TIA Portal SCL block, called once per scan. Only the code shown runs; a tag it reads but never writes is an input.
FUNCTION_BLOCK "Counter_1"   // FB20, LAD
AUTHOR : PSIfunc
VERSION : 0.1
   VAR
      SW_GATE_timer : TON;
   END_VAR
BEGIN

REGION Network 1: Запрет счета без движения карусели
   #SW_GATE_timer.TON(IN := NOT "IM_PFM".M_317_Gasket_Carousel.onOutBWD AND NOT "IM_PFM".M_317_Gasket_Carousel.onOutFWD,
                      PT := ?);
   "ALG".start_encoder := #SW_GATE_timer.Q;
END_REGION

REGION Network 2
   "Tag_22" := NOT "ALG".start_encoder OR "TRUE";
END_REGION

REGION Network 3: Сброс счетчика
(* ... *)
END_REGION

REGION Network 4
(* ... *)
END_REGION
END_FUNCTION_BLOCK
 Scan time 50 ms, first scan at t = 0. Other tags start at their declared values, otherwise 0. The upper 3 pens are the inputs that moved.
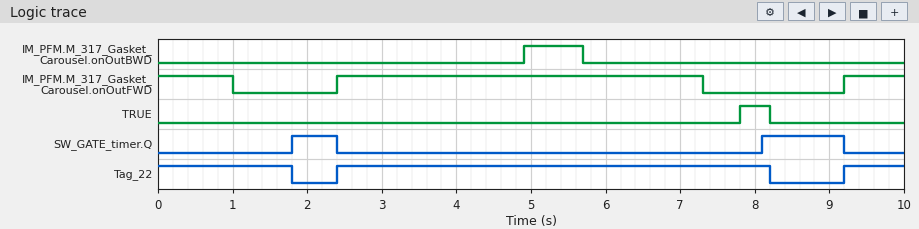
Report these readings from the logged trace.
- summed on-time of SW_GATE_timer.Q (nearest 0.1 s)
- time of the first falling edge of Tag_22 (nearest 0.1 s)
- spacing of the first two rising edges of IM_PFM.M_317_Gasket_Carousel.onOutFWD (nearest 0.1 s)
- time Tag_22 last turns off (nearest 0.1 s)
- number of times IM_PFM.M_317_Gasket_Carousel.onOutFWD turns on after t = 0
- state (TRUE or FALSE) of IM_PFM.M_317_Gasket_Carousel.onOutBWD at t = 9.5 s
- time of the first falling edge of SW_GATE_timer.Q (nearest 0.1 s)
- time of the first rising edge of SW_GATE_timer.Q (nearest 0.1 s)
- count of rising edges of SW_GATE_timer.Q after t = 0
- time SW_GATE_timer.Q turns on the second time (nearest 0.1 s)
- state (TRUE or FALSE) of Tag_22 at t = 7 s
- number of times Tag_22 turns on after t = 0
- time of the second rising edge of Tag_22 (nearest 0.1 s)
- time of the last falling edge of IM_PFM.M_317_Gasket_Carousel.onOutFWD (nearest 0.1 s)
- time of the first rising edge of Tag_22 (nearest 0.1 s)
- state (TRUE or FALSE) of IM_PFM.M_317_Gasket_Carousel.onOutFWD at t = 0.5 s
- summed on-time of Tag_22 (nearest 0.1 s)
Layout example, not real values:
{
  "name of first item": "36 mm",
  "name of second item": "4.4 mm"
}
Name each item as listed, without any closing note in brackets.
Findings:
{
  "summed on-time of SW_GATE_timer.Q": "1.7 s",
  "time of the first falling edge of Tag_22": "1.8 s",
  "spacing of the first two rising edges of IM_PFM.M_317_Gasket_Carousel.onOutFWD": "6.8 s",
  "time Tag_22 last turns off": "8.2 s",
  "number of times IM_PFM.M_317_Gasket_Carousel.onOutFWD turns on after t = 0": "2",
  "state (TRUE or FALSE) of IM_PFM.M_317_Gasket_Carousel.onOutBWD at t = 9.5 s": "FALSE",
  "time of the first falling edge of SW_GATE_timer.Q": "2.4 s",
  "time of the first rising edge of SW_GATE_timer.Q": "1.8 s",
  "count of rising edges of SW_GATE_timer.Q after t = 0": "2",
  "time SW_GATE_timer.Q turns on the second time": "8.1 s",
  "state (TRUE or FALSE) of Tag_22 at t = 7 s": "TRUE",
  "number of times Tag_22 turns on after t = 0": "2",
  "time of the second rising edge of Tag_22": "9.2 s",
  "time of the last falling edge of IM_PFM.M_317_Gasket_Carousel.onOutFWD": "7.3 s",
  "time of the first rising edge of Tag_22": "2.4 s",
  "state (TRUE or FALSE) of IM_PFM.M_317_Gasket_Carousel.onOutFWD at t = 0.5 s": "TRUE",
  "summed on-time of Tag_22": "8.4 s"
}
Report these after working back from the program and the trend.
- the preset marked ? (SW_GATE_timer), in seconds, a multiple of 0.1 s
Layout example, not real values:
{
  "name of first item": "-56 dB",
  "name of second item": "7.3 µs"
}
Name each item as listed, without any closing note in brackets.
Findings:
{
  "the preset marked ? (SW_GATE_timer), in seconds, a multiple of 0.1 s": "0.8 s"
}
